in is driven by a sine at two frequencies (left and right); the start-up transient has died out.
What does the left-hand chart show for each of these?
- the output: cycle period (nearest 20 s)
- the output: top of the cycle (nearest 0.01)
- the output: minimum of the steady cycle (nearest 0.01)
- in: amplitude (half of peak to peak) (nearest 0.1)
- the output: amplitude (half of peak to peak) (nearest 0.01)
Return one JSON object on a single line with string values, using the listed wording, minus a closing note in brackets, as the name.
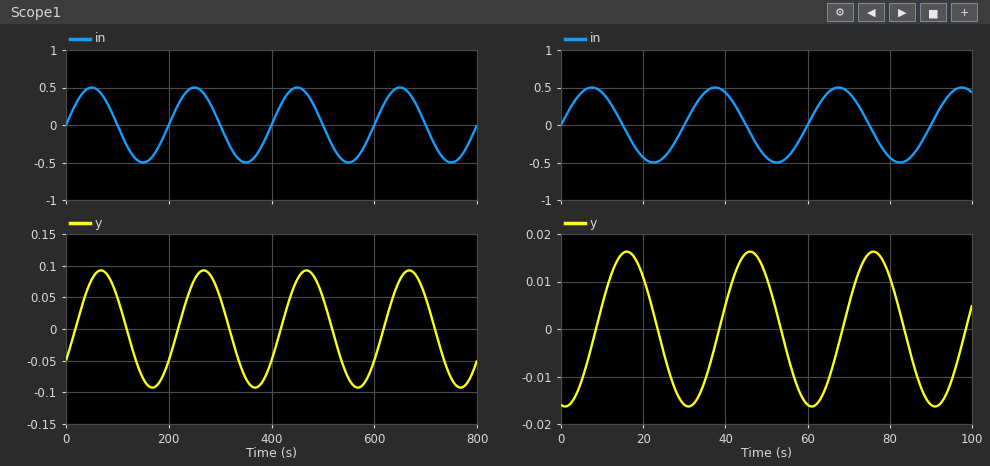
{"the output: cycle period": "200 s", "the output: top of the cycle": "0.09", "the output: minimum of the steady cycle": "-0.09", "in: amplitude (half of peak to peak)": "0.5", "the output: amplitude (half of peak to peak)": "0.09"}
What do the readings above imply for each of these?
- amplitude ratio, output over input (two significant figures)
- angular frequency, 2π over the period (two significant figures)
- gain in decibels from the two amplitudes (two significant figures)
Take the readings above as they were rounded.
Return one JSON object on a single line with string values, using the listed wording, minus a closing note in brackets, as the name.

{"amplitude ratio, output over input": "0.18", "angular frequency, 2π over the period": "0.031 rad/s", "gain in decibels from the two amplitudes": "-15 dB"}
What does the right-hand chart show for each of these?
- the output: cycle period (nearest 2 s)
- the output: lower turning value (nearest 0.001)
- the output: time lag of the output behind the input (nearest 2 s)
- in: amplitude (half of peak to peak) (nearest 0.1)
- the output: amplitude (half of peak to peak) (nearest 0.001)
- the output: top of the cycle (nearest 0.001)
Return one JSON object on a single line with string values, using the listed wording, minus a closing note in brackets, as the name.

{"the output: cycle period": "30 s", "the output: lower turning value": "-0.016", "the output: time lag of the output behind the input": "8 s", "in: amplitude (half of peak to peak)": "0.5", "the output: amplitude (half of peak to peak)": "0.016", "the output: top of the cycle": "0.016"}
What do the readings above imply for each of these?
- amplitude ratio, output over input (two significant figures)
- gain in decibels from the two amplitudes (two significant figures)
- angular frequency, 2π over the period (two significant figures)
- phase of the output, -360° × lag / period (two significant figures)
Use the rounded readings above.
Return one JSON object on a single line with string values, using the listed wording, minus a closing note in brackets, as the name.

{"amplitude ratio, output over input": "0.032", "gain in decibels from the two amplitudes": "-30 dB", "angular frequency, 2π over the period": "0.21 rad/s", "phase of the output, -360° × lag / period": "-96°"}
